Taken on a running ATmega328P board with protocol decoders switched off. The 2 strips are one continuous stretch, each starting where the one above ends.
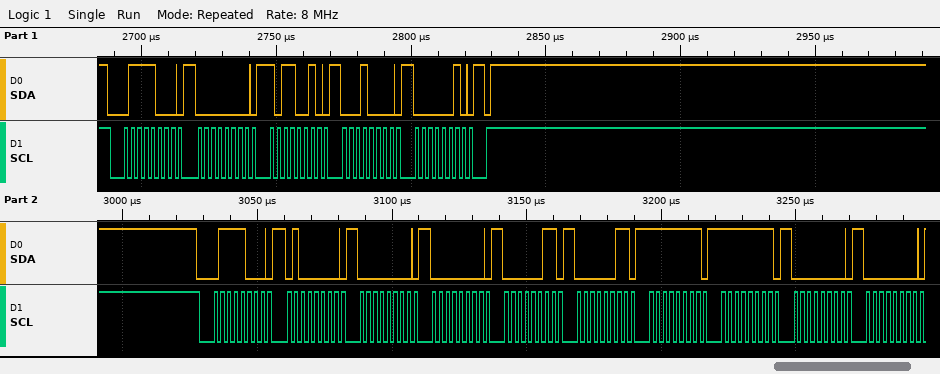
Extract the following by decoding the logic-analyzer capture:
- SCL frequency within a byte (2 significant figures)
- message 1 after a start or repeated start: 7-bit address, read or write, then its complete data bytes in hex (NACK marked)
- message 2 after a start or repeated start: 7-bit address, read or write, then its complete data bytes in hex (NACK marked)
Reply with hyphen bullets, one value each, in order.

- 400 kHz
- 0x3C write: 00 B2 10 02
- 0x3C write: 40 00 00 03 03 FF FF 00 00
